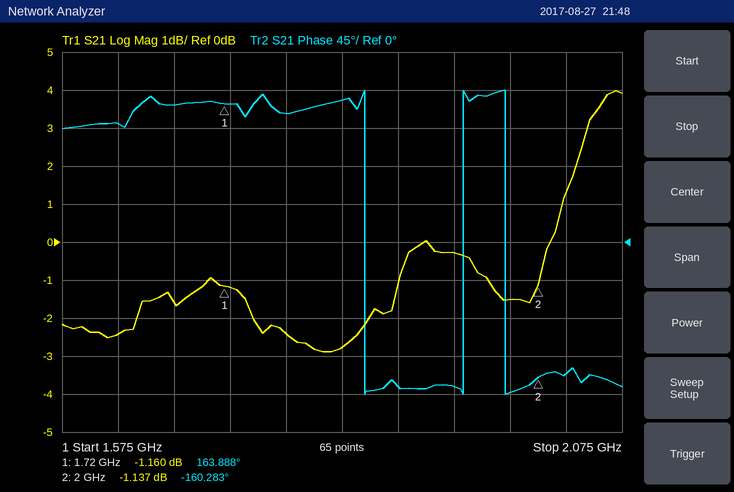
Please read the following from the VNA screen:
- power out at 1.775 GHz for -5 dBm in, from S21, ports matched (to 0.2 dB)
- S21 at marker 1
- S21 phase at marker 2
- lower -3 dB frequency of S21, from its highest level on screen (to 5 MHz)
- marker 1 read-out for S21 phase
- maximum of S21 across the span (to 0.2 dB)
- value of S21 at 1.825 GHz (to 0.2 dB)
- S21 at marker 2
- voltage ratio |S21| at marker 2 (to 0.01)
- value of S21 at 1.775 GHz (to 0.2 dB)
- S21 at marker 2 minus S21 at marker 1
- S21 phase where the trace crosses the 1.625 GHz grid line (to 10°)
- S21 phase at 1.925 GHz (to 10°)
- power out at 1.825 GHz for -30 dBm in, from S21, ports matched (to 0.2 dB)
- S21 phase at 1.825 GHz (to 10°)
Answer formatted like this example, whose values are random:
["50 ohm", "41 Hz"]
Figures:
["-7.4 dBm", "-1.160 dB", "-160.283°", "2.020 GHz", "163.888°", "4.0 dB", "-2.8 dB", "-1.137 dB", "0.88", "-2.4 dB", "0.023 dB", "140°", "-170°", "-32.8 dBm", "170°"]
